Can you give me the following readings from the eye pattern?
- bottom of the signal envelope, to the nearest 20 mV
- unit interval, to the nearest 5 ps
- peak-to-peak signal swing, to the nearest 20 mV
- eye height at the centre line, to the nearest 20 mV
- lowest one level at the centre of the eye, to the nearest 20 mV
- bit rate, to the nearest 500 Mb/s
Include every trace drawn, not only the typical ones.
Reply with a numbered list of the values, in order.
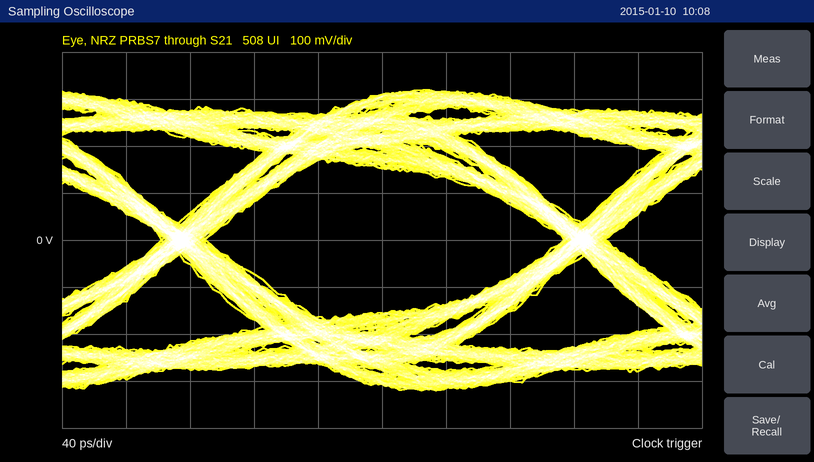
1. -320 mV
2. 250 ps
3. 640 mV
4. 300 mV
5. 160 mV
6. 4.0 Gb/s
